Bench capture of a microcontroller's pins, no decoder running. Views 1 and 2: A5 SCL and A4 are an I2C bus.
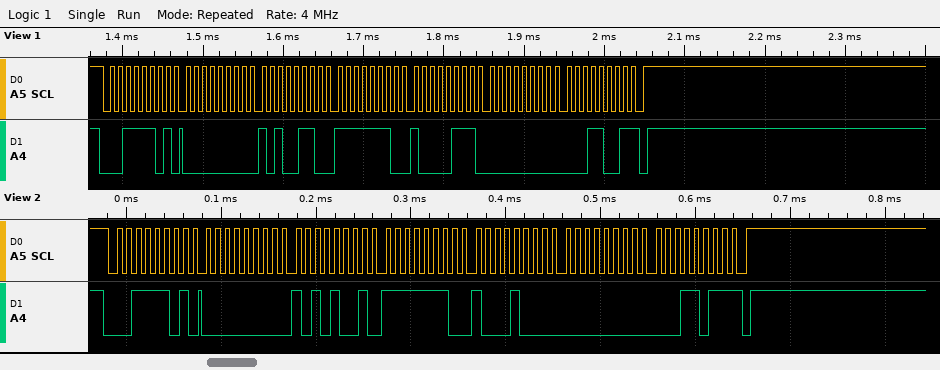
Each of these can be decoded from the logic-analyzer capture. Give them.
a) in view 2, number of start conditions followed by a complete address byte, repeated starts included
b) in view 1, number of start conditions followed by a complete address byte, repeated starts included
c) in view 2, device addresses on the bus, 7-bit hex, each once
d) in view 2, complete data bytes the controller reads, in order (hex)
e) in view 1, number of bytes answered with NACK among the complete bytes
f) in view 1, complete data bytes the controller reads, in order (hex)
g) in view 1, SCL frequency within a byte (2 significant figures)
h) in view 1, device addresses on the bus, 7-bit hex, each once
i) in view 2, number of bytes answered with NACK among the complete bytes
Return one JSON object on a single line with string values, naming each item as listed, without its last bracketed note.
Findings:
{"in view 2, number of start conditions followed by a complete address byte, repeated starts included": "1", "in view 1, number of start conditions followed by a complete address byte, repeated starts included": "1", "in view 2, device addresses on the bus, 7-bit hex, each once": "0x1E", "in view 2, complete data bytes the controller reads, in order": "00 A9 FE 88 00 1B", "in view 1, number of bytes answered with NACK among the complete bytes": "1", "in view 1, complete data bytes the controller reads, in order": "00 A6 FE 87 00 19", "in view 1, SCL frequency within a byte": "100 kHz", "in view 1, device addresses on the bus, 7-bit hex, each once": "0x1E", "in view 2, number of bytes answered with NACK among the complete bytes": "1"}
